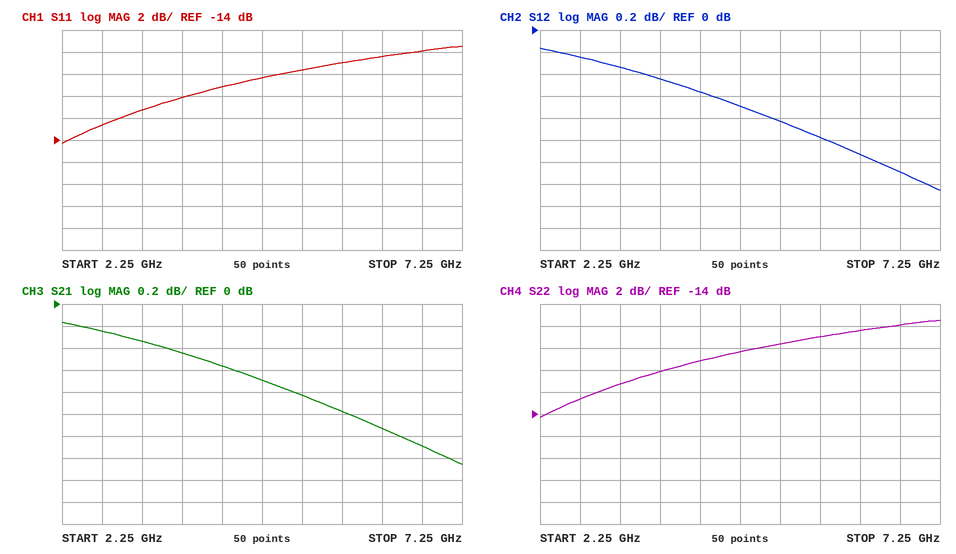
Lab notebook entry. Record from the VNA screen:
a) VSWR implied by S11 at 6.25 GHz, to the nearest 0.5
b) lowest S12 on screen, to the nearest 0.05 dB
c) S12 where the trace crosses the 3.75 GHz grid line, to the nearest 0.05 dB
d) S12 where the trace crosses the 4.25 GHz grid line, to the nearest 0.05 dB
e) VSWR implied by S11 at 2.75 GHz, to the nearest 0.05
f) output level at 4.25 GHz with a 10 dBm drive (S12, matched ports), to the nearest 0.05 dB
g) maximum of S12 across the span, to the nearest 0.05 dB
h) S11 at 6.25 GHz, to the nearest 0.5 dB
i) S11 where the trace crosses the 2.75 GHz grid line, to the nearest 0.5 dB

3.0
-1.45 dB
-0.45 dB
-0.55 dB
1.60
9.45 dBm
-0.15 dB
-6.5 dB
-12.5 dB
